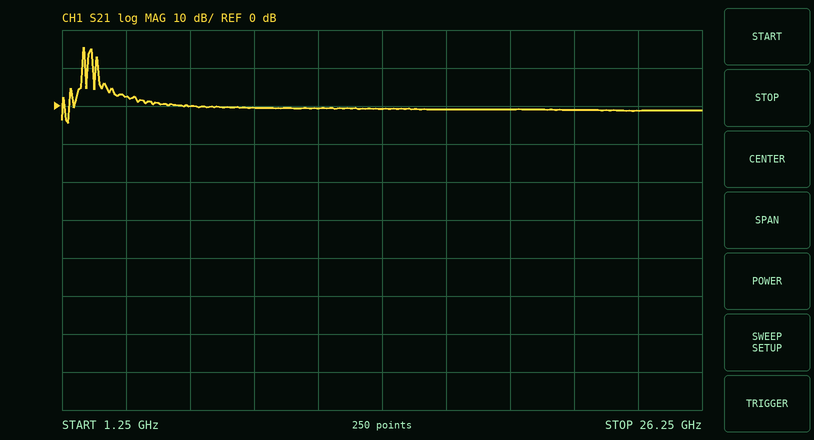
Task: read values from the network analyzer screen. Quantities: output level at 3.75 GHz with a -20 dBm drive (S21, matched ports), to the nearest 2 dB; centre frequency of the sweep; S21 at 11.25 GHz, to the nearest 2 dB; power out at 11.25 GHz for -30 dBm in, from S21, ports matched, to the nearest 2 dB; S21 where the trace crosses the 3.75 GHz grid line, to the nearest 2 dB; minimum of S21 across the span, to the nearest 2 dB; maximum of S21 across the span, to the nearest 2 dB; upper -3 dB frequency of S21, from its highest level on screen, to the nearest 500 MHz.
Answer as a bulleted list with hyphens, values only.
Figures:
- -18 dBm
- 13.75 GHz
- 0 dB
- -30 dBm
- 2 dB
- -4 dB
- 16 dB
- 2.0 GHz
